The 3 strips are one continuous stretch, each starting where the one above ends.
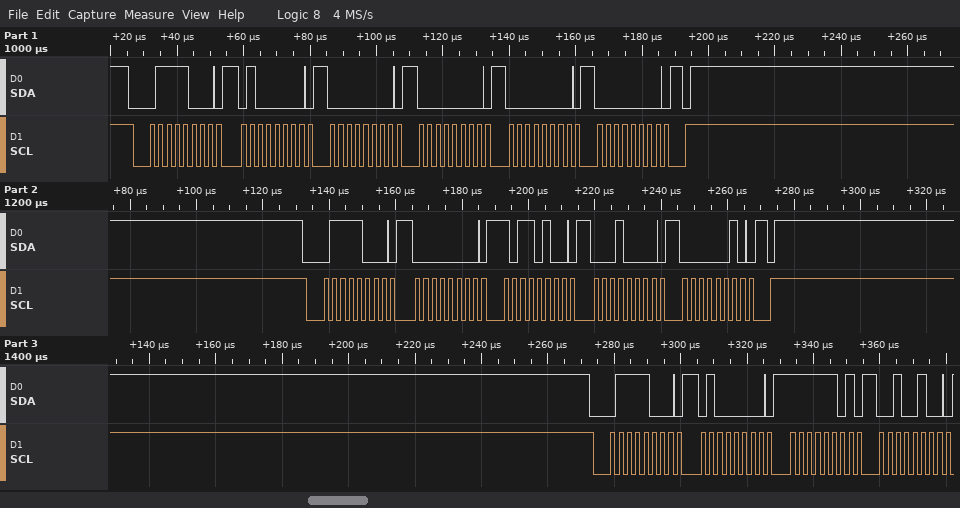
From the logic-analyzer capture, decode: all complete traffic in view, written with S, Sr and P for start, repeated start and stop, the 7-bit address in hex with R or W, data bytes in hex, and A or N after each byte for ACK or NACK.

S 3CW A 40 A 00 A 00 A 00 A 00 A P S 3CW A 00 A B4 A 10 A 02 A P S 3CW A 40 A FD A 24 A
